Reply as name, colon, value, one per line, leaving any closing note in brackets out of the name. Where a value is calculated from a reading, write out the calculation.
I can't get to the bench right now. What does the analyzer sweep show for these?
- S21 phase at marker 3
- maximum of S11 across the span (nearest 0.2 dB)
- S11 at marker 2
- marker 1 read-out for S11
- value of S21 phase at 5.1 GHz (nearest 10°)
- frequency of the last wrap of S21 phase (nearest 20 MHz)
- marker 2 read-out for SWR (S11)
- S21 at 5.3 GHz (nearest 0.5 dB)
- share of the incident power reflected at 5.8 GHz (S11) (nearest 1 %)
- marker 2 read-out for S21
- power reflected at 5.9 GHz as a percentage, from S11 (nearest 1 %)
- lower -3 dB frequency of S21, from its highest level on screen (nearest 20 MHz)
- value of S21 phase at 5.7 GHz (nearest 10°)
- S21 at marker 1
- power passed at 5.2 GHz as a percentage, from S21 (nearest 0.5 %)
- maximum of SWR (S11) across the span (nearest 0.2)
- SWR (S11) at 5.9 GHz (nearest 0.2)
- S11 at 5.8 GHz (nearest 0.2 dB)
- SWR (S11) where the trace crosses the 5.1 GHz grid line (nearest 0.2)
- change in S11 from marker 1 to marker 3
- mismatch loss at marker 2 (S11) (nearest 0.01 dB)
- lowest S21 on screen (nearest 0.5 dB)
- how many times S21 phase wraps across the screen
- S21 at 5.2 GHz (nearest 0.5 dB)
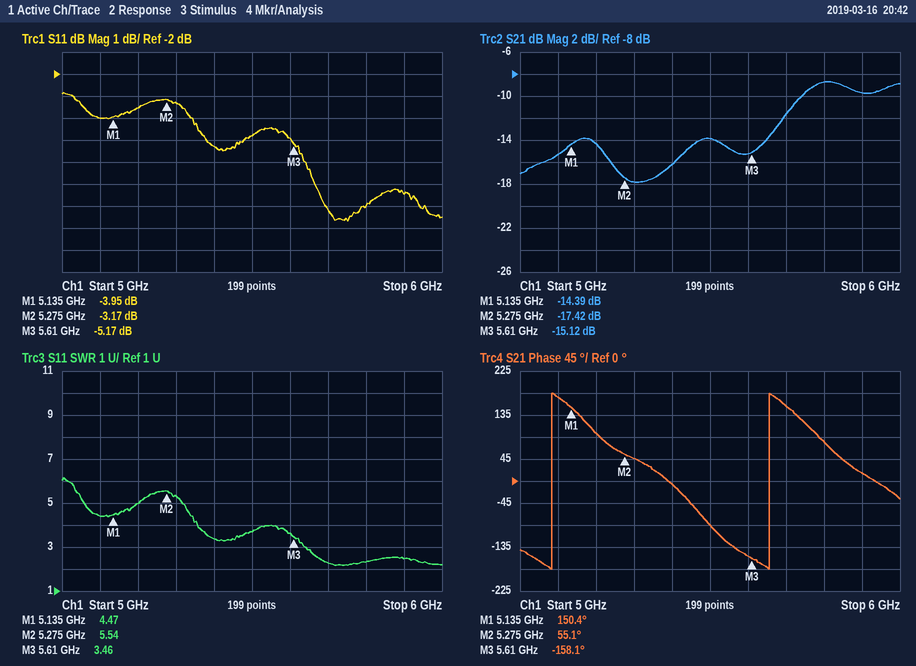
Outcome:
S21 phase at marker 3: -158.1°
maximum of S11 across the span: -2.8 dB
S11 at marker 2: -3.17 dB
marker 1 read-out for S11: -3.95 dB
value of S21 phase at 5.1 GHz: 170°
frequency of the last wrap of S21 phase: 5.66 GHz
marker 2 read-out for SWR: 5.54
S21 at 5.3 GHz: -18.0 dB
share of the incident power reflected at 5.8 GHz (S11): 10^(-8/10) ≈ 16 %
marker 2 read-out for S21: -17.42 dB
power reflected at 5.9 GHz as a percentage, from S11: 10^(-7.4/10) ≈ 18 %
lower -3 dB frequency of S21, from its highest level on screen: 5.70 GHz
value of S21 phase at 5.7 GHz: 150°
S21 at marker 1: -14.39 dB
power passed at 5.2 GHz as a percentage, from S21: 10^(-14.5/10) ≈ 3.5 %
maximum of SWR (S11) across the span: 6.2
SWR (S11) at 5.9 GHz: 2.4
S11 at 5.8 GHz: -8.0 dB
SWR (S11) where the trace crosses the 5.1 GHz grid line: 4.4
change in S11 from marker 1 to marker 3: -5.17 − (-3.95) = -1.22 dB
mismatch loss at marker 2 (S11): −10 log10(1 − 10^(-3.17/10)) ≈ 2.86 dB
lowest S21 on screen: -18.0 dB
how many times S21 phase wraps across the screen: 2
S21 at 5.2 GHz: -14.5 dB
